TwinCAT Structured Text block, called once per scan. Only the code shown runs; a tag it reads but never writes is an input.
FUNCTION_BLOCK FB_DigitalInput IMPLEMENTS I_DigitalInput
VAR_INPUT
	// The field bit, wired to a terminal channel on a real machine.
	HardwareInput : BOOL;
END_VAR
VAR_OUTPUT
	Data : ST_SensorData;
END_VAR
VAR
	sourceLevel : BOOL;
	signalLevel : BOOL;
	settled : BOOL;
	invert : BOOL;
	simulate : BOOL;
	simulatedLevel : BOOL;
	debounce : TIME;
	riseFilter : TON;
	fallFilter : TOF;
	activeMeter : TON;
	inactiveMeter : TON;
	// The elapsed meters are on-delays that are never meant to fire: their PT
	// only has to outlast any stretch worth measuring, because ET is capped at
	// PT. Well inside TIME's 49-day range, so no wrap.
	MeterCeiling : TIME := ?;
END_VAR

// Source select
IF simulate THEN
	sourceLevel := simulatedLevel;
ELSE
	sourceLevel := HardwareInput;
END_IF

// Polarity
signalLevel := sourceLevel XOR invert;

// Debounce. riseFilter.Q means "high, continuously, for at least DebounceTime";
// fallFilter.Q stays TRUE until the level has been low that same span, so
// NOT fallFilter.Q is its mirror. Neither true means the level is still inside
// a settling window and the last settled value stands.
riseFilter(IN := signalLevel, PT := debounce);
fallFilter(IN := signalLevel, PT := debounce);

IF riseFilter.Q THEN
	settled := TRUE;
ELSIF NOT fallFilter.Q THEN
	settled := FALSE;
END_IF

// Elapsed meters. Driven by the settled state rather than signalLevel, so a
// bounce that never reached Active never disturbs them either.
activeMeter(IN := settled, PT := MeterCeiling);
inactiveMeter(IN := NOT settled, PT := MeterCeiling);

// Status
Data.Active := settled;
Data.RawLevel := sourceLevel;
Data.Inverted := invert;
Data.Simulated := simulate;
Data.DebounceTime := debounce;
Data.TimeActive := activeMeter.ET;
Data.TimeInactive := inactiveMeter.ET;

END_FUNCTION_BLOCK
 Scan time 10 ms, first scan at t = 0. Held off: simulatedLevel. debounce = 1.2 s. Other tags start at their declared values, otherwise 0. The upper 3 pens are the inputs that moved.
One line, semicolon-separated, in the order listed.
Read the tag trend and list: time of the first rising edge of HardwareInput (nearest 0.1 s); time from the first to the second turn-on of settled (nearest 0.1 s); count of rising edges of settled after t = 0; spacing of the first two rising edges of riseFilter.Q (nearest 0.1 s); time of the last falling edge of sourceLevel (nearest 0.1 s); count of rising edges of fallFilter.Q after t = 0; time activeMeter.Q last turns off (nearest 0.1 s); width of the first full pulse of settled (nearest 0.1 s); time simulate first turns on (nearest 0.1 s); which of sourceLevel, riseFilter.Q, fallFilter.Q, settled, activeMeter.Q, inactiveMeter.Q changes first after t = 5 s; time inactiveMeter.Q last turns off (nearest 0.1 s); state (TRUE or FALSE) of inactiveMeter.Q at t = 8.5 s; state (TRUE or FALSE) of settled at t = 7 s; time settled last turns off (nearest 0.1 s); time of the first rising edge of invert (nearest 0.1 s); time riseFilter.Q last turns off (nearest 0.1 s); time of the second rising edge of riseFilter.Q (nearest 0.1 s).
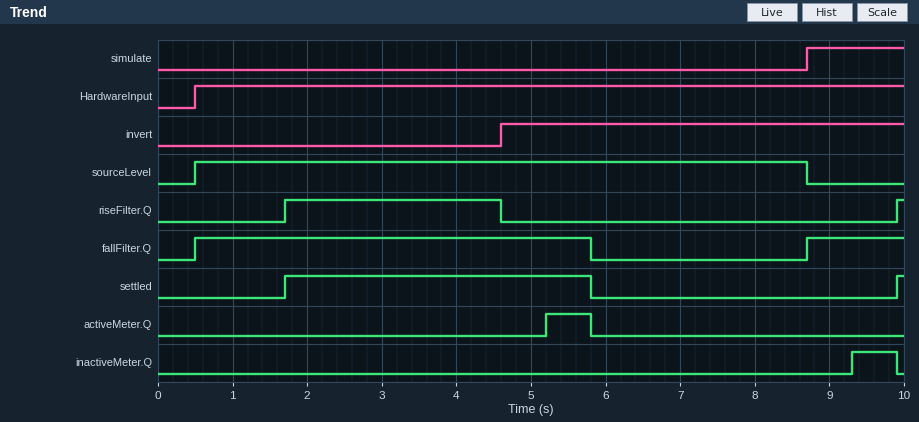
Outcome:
0.5 s; 8.2 s; 2; 8.2 s; 8.7 s; 2; 5.8 s; 4.1 s; 8.7 s; activeMeter.Q; 9.9 s; FALSE; FALSE; 5.8 s; 4.6 s; 4.6 s; 9.9 s
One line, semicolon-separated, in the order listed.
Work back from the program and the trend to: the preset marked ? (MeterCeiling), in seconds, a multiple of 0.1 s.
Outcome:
3.5 s
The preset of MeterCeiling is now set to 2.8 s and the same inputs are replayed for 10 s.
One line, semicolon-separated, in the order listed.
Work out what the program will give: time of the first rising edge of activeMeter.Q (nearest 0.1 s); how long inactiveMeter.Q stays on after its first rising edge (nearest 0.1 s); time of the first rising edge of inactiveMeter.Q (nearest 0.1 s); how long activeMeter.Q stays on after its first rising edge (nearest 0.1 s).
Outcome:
4.5 s; 1.3 s; 8.6 s; 1.3 s
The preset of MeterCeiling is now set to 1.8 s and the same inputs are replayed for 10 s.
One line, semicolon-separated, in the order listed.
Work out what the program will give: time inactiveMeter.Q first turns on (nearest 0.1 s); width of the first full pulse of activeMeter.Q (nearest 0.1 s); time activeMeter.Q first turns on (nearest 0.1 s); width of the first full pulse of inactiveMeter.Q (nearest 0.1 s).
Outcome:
7.6 s; 2.3 s; 3.5 s; 2.3 s
